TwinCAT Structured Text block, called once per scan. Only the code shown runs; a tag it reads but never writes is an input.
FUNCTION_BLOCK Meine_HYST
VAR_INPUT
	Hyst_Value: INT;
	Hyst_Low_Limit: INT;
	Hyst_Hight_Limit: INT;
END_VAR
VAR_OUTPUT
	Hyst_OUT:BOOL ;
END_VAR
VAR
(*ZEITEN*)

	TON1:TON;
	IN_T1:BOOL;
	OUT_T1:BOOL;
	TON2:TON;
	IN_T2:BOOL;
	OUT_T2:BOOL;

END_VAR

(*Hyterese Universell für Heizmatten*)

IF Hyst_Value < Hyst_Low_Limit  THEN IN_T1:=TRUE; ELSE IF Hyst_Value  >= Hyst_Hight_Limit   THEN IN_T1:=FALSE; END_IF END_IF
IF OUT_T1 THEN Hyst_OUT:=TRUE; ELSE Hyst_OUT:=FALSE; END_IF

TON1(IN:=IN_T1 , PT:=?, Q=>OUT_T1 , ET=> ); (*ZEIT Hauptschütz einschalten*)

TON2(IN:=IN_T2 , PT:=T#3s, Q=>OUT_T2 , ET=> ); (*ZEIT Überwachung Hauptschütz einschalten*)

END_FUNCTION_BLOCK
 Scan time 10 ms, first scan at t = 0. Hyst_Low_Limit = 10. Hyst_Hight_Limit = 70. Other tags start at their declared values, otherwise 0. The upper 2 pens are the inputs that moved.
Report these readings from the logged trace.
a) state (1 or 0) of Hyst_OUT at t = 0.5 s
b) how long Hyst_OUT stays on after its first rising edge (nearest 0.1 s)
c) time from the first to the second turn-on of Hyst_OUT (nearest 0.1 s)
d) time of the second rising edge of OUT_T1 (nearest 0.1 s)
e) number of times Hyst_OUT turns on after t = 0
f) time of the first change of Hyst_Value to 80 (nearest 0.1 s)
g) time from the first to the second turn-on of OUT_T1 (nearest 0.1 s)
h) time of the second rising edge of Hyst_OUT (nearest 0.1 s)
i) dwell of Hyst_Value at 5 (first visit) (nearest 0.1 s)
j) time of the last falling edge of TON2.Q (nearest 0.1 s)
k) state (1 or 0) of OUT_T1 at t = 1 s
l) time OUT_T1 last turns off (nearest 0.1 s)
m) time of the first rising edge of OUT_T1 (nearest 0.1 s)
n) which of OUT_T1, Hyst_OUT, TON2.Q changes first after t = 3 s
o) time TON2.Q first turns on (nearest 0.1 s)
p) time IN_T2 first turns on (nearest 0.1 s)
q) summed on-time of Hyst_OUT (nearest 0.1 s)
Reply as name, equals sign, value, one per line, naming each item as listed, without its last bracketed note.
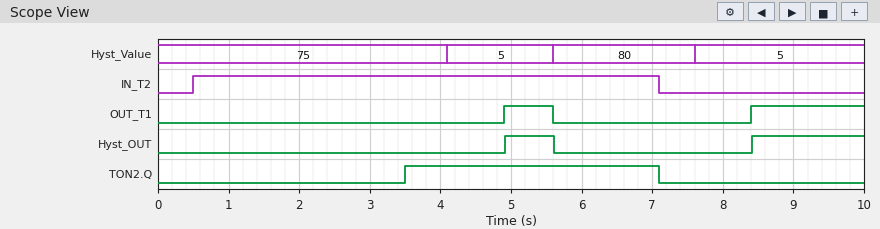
state (1 or 0) of Hyst_OUT at t = 0.5 s = 0
how long Hyst_OUT stays on after its first rising edge = 0.7 s
time from the first to the second turn-on of Hyst_OUT = 3.5 s
time of the second rising edge of OUT_T1 = 8.4 s
number of times Hyst_OUT turns on after t = 0 = 2
time of the first change of Hyst_Value to 80 = 5.6 s
time from the first to the second turn-on of OUT_T1 = 3.5 s
time of the second rising edge of Hyst_OUT = 8.4 s
dwell of Hyst_Value at 5 (first visit) = 1.5 s
time of the last falling edge of TON2.Q = 7.1 s
state (1 or 0) of OUT_T1 at t = 1 s = 0
time OUT_T1 last turns off = 5.6 s
time of the first rising edge of OUT_T1 = 4.9 s
which of OUT_T1, Hyst_OUT, TON2.Q changes first after t = 3 s = TON2.Q
time TON2.Q first turns on = 3.5 s
time IN_T2 first turns on = 0.5 s
summed on-time of Hyst_OUT = 2.3 s
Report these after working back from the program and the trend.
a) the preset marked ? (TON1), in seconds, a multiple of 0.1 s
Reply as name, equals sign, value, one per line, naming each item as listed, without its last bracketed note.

the preset marked ? (TON1), in seconds, a multiple of 0.1 s = 0.8 s
